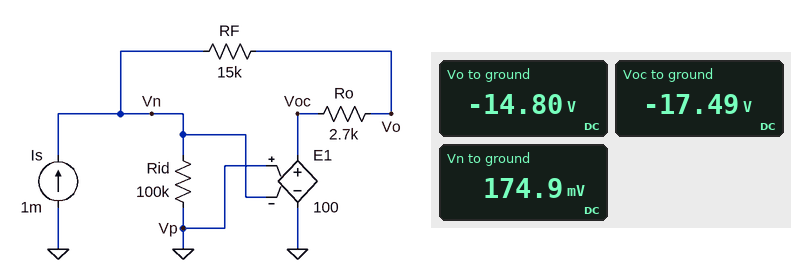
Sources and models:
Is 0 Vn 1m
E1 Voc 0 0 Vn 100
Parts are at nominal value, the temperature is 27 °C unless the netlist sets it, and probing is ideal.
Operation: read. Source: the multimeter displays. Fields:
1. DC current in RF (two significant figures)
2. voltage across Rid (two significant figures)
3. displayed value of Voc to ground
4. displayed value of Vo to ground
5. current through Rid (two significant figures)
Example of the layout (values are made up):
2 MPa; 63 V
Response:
1.0 mA; 170 mV; -17.49 V; -14.80 V; 1.7 µA
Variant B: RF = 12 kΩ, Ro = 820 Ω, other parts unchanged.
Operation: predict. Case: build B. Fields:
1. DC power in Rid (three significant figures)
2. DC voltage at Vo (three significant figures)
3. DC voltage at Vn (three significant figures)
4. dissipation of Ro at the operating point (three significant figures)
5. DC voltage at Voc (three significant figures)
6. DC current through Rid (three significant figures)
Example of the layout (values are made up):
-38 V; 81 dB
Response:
161 nW; -11.9 V; 127 mV; 818 µW; -12.7 V; 1.27 µA
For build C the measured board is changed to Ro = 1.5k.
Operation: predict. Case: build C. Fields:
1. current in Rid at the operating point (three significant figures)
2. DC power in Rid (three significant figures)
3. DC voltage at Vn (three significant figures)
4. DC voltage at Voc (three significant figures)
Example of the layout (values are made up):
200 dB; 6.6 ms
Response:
1.63 µA; 266 nW; 163 mV; -16.3 V
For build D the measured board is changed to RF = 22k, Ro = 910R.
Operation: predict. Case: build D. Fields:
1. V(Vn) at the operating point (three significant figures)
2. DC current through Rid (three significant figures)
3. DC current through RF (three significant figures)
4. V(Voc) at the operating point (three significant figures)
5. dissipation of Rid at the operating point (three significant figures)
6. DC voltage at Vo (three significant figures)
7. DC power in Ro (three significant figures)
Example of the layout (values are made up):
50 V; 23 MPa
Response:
226 mV; 2.26 µA; 998 µA; -22.6 V; 512 nW; -21.7 V; 906 µW
